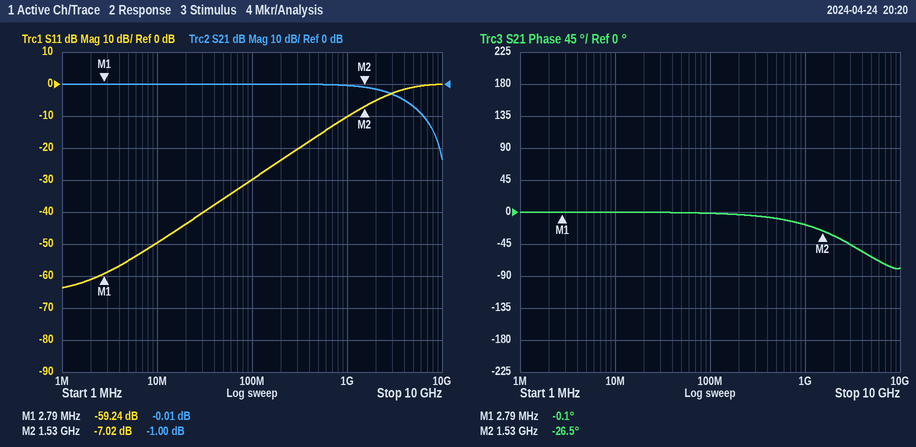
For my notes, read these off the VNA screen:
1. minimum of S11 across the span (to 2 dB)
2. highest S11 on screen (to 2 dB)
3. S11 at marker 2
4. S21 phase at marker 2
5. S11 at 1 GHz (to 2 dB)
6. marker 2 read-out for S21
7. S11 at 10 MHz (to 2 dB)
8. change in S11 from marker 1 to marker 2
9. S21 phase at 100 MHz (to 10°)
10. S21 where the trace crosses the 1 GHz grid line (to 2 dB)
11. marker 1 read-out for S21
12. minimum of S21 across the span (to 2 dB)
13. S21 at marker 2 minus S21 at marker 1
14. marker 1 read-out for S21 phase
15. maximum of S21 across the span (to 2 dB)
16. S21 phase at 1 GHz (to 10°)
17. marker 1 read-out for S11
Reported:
-64 dB
0 dB
-7.02 dB
-26.5°
-10 dB
-1.00 dB
-50 dB
52.22 dB
0°
0 dB
-0.01 dB
-24 dB
-0.99 dB
-0.1°
0 dB
-20°
-59.24 dB
